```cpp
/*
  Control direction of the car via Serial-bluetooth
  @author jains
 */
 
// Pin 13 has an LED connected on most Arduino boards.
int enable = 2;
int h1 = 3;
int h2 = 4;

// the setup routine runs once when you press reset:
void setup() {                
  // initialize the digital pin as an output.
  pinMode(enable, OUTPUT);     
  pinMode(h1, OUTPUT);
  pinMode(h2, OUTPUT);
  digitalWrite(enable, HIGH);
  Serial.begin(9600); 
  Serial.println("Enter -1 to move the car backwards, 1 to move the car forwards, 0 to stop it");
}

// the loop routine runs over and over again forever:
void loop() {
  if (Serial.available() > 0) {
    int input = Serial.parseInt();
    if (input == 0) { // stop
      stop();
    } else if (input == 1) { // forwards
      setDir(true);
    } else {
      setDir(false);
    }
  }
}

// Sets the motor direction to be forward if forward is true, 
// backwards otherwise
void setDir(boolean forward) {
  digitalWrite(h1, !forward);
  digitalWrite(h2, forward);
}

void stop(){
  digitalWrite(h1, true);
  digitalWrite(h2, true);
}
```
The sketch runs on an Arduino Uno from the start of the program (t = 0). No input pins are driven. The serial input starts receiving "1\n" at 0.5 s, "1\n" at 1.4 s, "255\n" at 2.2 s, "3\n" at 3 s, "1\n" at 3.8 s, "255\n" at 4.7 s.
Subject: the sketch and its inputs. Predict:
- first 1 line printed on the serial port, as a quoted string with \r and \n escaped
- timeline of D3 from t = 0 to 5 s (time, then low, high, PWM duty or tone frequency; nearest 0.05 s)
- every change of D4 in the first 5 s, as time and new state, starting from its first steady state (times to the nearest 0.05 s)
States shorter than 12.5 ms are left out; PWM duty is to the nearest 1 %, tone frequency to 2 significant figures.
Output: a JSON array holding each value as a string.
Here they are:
["\"Enter -1 to move the car backwards, 1 to move the car forwards, 0 to stop it\\r\\n\"", "0 s low; 2.2 s high; 3.8 s low; 4.7 s high", "0 s low; 0.5 s high; 2.2 s low; 3.8 s high; 4.7 s low"]
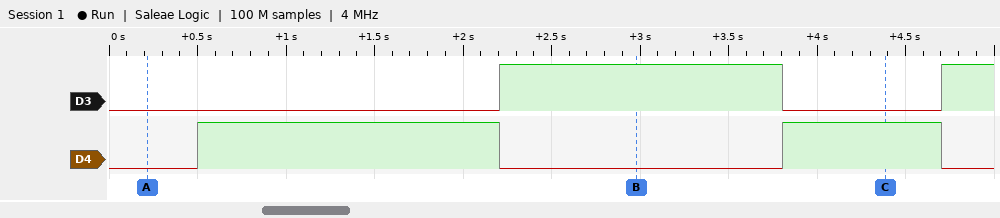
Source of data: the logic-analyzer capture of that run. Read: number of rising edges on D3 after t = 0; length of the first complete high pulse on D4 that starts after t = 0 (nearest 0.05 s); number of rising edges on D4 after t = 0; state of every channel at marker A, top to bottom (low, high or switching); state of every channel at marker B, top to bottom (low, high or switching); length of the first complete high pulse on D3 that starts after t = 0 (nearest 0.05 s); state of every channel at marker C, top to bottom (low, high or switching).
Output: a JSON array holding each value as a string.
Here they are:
["2", "1.70 s", "2", "D3 low, D4 low", "D3 high, D4 low", "1.60 s", "D3 low, D4 high"]
